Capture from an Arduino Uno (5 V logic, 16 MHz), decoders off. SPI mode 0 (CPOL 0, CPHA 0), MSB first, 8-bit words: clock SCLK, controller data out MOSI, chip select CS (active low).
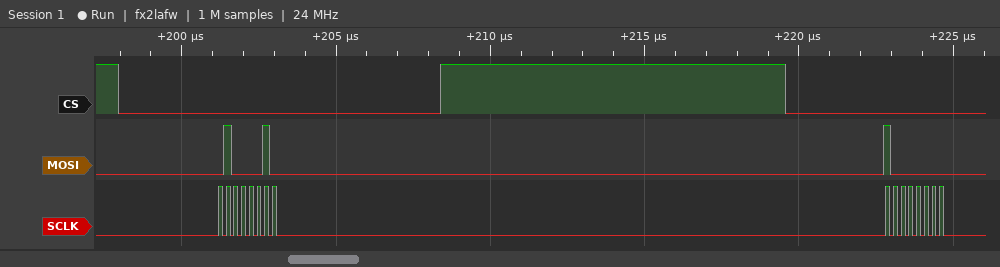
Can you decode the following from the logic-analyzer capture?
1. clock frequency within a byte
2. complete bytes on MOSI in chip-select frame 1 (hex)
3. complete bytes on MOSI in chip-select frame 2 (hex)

4 MHz
42
80
